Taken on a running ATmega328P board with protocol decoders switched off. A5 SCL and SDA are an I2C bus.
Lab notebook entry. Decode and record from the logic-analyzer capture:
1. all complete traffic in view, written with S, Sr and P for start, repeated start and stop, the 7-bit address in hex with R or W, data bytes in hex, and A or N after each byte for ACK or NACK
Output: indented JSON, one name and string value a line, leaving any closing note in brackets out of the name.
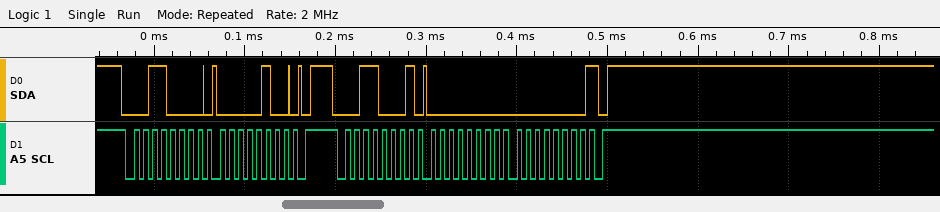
{
  "all complete traffic in view, written with S, Sr and P for start, repeated start and stop, the 7-bit address in hex with R or W, data bytes in hex, and A or N after each byte for ACK or NACK": "S 18W A 04 A P S 18R A 00 A 00 N P"
}
